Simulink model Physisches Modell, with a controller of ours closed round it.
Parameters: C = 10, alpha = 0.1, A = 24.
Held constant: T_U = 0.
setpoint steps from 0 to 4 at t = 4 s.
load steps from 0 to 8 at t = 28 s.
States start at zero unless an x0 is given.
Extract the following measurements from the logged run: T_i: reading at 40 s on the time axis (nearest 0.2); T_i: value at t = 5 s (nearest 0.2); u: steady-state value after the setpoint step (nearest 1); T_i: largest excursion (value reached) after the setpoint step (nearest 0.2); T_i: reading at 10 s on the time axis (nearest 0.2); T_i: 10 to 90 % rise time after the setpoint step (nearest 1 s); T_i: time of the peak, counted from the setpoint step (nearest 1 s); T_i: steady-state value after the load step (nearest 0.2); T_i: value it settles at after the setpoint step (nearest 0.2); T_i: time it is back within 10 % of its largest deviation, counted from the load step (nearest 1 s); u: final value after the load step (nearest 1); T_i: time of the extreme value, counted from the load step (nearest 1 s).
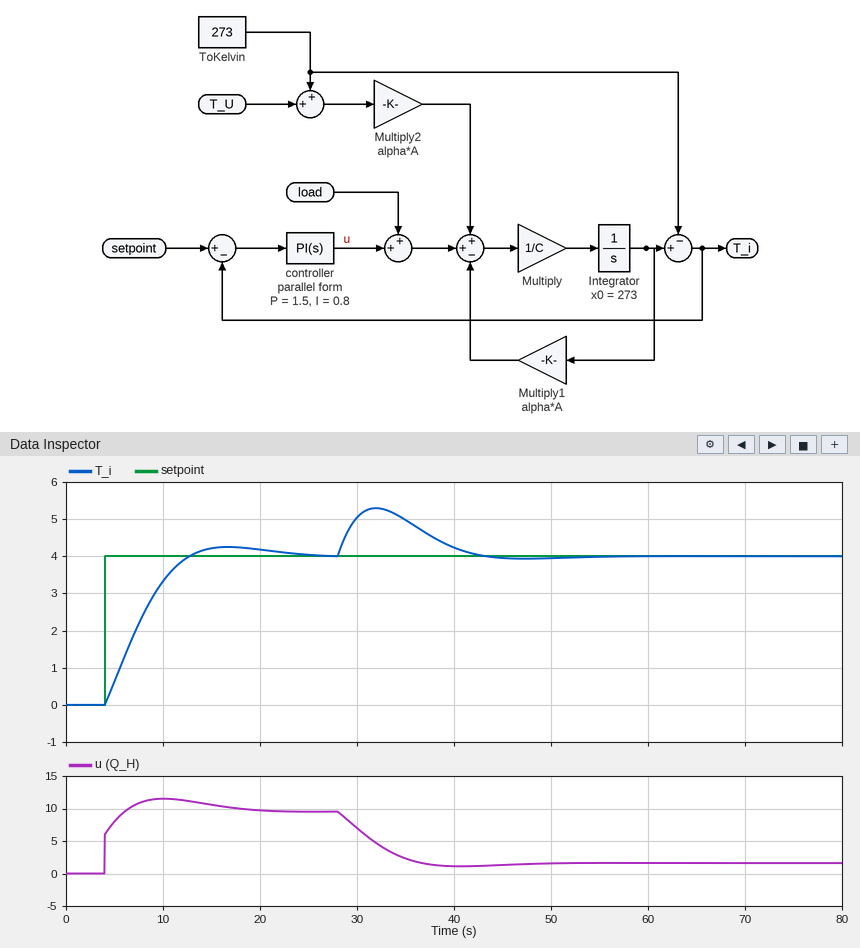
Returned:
4.2
0.6
10
4.2
3.4
6 s
13 s
4.0
4.0
13 s
2
4 s
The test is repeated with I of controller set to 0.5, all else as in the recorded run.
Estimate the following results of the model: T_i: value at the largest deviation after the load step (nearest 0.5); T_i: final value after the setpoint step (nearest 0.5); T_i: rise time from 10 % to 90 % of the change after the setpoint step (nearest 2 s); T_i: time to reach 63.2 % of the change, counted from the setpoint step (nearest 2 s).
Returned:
5.5
4.0
10 s
6 s
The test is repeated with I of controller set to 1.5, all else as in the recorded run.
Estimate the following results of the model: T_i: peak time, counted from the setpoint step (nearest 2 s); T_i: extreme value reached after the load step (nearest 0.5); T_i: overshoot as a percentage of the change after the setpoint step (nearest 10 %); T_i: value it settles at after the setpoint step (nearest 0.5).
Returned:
8 s
5.0
20 %
4.0
